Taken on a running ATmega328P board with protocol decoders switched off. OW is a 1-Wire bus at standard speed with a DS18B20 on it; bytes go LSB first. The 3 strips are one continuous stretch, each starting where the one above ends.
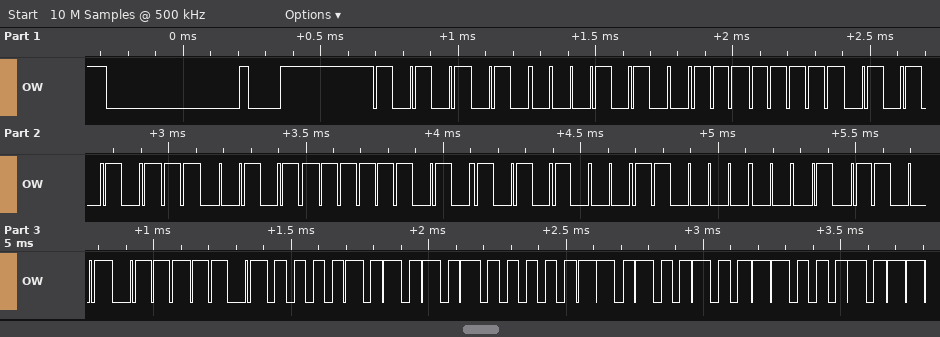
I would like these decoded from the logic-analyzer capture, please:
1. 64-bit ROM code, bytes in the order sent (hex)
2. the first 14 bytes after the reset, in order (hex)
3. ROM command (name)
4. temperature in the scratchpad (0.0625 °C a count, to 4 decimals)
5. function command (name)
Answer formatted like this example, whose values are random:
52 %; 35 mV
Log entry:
28 FF AA D3 5F 15 03 9A; 55 28 FF AA D3 5F 15 03 9A BE 50 05 4B 46; Match ROM; 85.0000 °C; Read Scratchpad
